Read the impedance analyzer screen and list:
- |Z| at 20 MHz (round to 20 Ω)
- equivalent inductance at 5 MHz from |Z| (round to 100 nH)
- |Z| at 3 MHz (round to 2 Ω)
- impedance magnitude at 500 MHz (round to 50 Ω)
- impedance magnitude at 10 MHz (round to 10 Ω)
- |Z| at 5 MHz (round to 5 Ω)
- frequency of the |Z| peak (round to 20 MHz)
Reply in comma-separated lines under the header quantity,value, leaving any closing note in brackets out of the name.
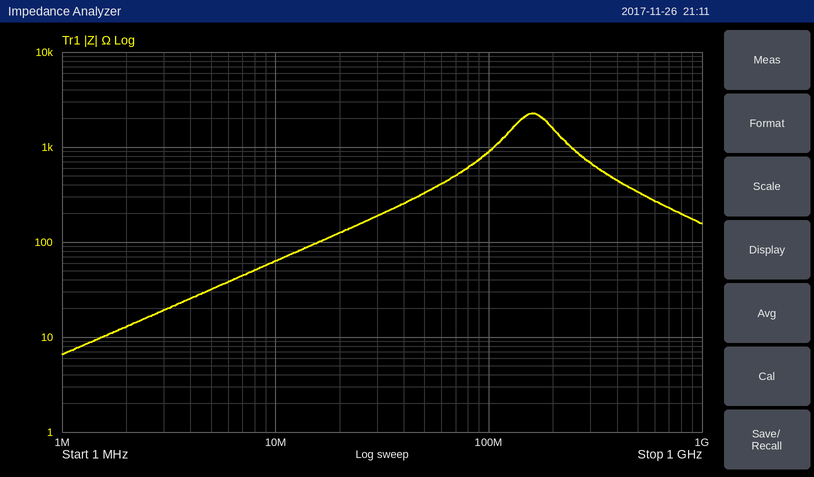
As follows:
quantity,value
|Z| at 20 MHz,120 Ω
equivalent inductance at 5 MHz from |Z|,1.0 µH
|Z| at 3 MHz,20 Ω
impedance magnitude at 500 MHz,350 Ω
impedance magnitude at 10 MHz,60 Ω
|Z| at 5 MHz,30 Ω
frequency of the |Z| peak,160 MHz
